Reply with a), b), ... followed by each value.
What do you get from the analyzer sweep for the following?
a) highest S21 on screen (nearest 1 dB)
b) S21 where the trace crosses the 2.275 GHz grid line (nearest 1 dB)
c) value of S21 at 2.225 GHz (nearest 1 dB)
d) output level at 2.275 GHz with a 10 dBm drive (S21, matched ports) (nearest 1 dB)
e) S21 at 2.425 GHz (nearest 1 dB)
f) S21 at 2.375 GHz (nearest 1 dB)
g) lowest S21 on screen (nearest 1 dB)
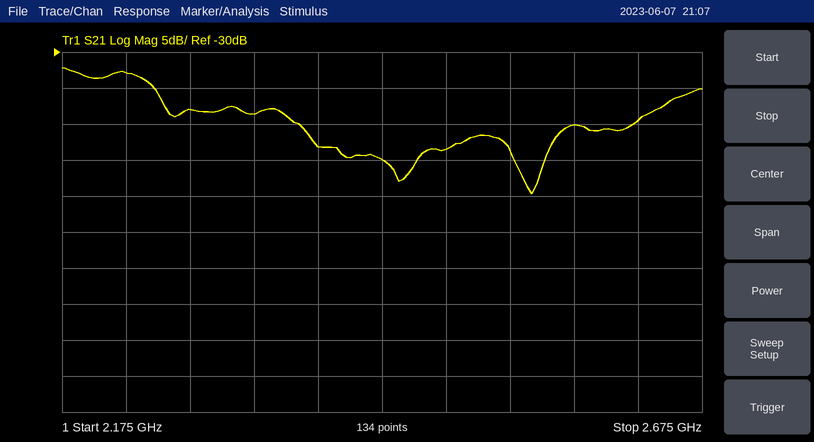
a) -32 dB
b) -38 dB
c) -33 dB
d) -28 dBm
e) -45 dB
f) -43 dB
g) -50 dB
